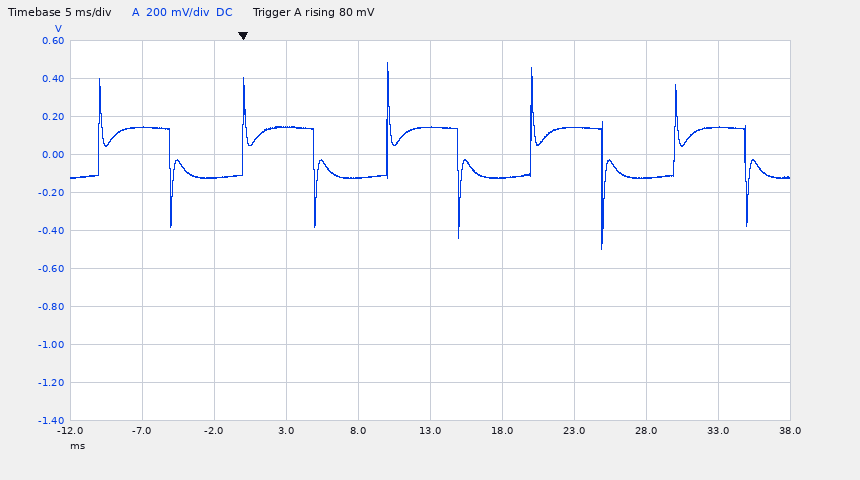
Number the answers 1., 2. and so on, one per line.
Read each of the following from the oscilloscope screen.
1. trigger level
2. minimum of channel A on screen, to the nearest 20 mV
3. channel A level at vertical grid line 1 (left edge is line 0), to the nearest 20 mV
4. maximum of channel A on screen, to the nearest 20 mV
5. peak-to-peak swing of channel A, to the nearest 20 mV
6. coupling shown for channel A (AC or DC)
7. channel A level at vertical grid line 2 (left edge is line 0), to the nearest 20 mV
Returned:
1. 80 mV
2. -500 mV
3. 140 mV
4. 480 mV
5. 980 mV
6. DC
7. -120 mV
